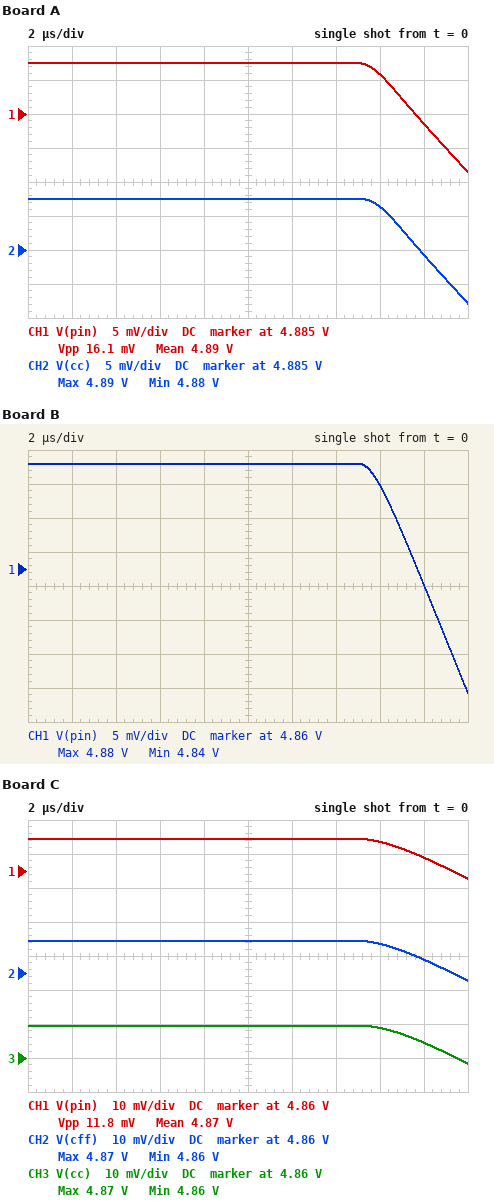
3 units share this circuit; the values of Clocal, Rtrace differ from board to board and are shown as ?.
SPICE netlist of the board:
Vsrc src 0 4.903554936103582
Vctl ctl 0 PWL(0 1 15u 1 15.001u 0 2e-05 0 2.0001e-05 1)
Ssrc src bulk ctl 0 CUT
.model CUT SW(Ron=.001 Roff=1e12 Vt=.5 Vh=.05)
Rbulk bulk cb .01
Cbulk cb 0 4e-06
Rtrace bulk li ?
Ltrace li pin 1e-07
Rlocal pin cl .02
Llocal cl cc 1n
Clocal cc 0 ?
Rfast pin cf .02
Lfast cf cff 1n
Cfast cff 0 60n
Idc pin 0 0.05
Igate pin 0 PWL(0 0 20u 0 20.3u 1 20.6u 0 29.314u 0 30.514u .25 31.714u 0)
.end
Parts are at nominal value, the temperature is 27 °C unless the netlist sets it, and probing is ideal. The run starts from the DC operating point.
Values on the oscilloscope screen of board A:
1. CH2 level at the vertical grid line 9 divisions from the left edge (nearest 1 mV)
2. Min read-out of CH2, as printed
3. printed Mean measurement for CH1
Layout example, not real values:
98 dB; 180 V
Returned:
4.884 V; 4.88 V; 4.89 V
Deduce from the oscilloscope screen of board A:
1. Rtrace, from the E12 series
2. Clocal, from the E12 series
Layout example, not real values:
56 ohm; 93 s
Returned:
0.22 Ω; 10 µF
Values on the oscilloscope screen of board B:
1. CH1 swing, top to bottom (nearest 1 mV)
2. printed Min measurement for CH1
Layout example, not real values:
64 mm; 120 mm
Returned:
34 mV; 4.84 V
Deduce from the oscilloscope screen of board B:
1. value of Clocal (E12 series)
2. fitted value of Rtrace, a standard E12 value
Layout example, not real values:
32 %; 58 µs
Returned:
2.2 µF; 0.56 Ω
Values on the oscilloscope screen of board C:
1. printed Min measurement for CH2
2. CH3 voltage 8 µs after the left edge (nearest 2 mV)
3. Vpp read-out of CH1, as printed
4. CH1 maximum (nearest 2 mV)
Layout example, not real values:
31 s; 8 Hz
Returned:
4.86 V; 4.870 V; 11.8 mV; 4.870 V
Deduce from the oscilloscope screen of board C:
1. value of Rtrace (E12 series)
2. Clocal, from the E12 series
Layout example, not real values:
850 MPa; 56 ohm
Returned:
0.68 Ω; 10 µF
